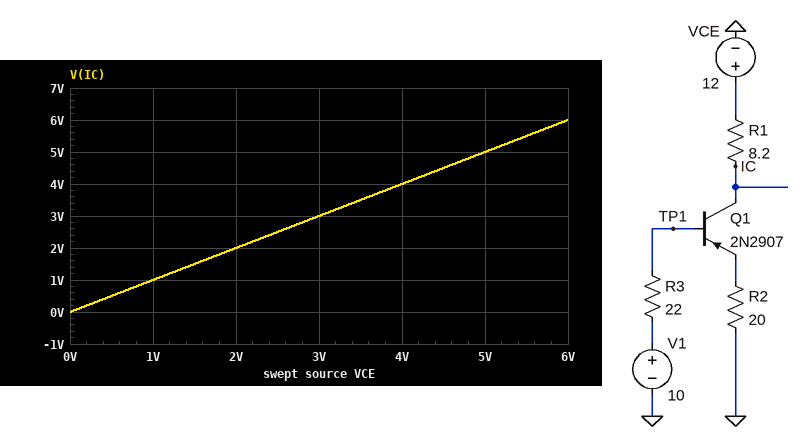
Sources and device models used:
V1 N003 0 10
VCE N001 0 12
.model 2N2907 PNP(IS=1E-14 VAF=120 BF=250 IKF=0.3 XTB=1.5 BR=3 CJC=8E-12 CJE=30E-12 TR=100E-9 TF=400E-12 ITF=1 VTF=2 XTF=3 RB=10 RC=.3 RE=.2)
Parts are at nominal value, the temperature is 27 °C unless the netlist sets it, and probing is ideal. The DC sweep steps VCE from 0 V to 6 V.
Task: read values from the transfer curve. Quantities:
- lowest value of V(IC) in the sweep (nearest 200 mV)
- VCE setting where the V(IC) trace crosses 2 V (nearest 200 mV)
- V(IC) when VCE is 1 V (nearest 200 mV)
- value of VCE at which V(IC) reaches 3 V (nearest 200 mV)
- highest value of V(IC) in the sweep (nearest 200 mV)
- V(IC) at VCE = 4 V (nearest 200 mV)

0 V
2.0 V
1.0 V
3.0 V
6.0 V
4.0 V
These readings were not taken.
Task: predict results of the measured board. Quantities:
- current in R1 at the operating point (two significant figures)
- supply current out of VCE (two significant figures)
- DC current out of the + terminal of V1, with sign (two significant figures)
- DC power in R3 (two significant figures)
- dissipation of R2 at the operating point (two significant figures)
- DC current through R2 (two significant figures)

75 mA
75 mA
-19 mA
7.8 mW
63 mW
56 mA
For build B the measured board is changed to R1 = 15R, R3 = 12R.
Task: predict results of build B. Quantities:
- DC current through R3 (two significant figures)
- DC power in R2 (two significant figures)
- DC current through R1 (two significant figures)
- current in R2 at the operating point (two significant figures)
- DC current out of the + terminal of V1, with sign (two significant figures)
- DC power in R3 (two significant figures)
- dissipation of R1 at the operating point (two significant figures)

15 mA
40 mW
60 mA
45 mA
-15 mA
2.7 mW
54 mW
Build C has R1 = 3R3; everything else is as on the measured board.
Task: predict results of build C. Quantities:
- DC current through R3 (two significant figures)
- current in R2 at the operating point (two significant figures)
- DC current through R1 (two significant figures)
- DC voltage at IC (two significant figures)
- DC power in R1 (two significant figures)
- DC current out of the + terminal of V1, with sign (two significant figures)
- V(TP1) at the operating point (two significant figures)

27 mA
79 mA
110 mA
12 V
37 mW
-27 mA
11 V
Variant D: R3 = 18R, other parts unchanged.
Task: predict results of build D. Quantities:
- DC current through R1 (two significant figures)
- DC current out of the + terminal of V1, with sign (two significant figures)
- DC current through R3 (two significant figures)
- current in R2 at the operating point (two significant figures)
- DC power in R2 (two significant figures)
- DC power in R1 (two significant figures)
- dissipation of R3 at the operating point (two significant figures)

80 mA
-20 mA
20 mA
60 mA
71 mW
52 mW
7.2 mW
